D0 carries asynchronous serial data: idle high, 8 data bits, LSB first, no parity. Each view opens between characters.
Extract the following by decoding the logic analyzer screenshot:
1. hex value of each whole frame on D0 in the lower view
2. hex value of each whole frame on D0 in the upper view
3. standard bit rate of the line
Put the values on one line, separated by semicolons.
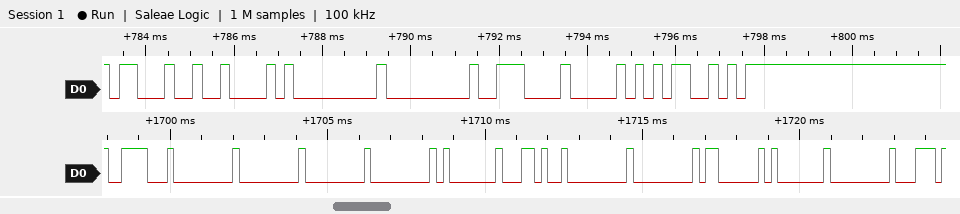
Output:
1E, 00, 00, 00, 00, 01, 2C, 00, 00, 03, 01, 00; 23, 42, 00, 00, 0E, 50, 53; 4800 baud
